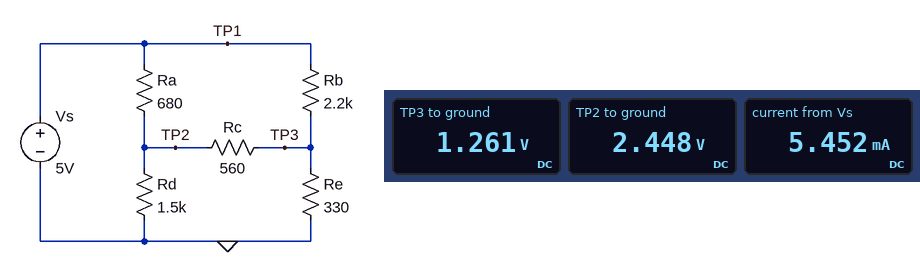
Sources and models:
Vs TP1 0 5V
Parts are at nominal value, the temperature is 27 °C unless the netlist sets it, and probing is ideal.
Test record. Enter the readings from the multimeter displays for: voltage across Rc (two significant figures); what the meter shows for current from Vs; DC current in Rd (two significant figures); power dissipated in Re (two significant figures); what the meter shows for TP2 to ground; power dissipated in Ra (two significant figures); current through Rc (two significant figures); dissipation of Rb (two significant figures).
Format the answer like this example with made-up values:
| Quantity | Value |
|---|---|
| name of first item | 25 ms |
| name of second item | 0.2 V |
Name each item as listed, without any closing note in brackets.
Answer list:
| Quantity | Value |
|---|---|
| voltage across Rc | 1.2 V |
| what the meter shows for current from Vs | 5.452 mA |
| DC current in Rd | 1.6 mA |
| power dissipated in Re | 4.8 mW |
| what the meter shows for TP2 to ground | 2.448 V |
| power dissipated in Ra | 9.6 mW |
| current through Rc | 2.1 mA |
| dissipation of Rb | 6.4 mW |
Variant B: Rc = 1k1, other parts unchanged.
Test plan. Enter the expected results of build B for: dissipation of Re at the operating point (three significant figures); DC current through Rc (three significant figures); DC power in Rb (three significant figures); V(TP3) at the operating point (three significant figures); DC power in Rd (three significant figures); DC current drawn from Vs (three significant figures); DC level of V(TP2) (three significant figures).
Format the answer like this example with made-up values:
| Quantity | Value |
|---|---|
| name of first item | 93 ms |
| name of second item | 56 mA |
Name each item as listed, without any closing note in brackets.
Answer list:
| Quantity | Value |
|---|---|
| dissipation of Re at the operating point | 3.56 mW |
| DC current through Rc | 1.50 mA |
| DC power in Rb | 6.97 mW |
| V(TP3) at the operating point | 1.08 V |
| DC power in Rd | 4.99 mW |
| DC current drawn from Vs | 5.11 mA |
| DC level of V(TP2) | 2.74 V |
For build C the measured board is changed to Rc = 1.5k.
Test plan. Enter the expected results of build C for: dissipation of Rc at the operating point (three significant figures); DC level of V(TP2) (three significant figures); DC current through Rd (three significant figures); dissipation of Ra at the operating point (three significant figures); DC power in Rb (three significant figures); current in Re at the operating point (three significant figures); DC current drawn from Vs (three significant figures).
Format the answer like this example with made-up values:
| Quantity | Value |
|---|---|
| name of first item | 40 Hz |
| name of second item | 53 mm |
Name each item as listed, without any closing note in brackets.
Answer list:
| Quantity | Value |
|---|---|
| dissipation of Rc at the operating point | 2.29 mW |
| DC level of V(TP2) | 2.86 V |
| DC current through Rd | 1.91 mA |
| dissipation of Ra at the operating point | 6.72 mW |
| DC power in Rb | 7.25 mW |
| current in Re at the operating point | 3.05 mA |
| DC current drawn from Vs | 4.96 mA |
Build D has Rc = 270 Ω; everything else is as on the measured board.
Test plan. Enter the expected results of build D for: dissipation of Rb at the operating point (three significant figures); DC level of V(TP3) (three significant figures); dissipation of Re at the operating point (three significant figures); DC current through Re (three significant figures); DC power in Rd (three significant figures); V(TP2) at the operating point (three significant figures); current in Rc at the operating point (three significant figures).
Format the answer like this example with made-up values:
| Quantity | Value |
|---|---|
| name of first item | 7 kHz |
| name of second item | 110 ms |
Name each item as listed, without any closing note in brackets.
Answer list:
| Quantity | Value |
|---|---|
| dissipation of Rb at the operating point | 5.78 mW |
| DC level of V(TP3) | 1.43 V |
| dissipation of Re at the operating point | 6.22 mW |
| DC current through Re | 4.34 mA |
| DC power in Rd | 3.13 mW |
| V(TP2) at the operating point | 2.17 V |
| current in Rc at the operating point | 2.72 mA |
